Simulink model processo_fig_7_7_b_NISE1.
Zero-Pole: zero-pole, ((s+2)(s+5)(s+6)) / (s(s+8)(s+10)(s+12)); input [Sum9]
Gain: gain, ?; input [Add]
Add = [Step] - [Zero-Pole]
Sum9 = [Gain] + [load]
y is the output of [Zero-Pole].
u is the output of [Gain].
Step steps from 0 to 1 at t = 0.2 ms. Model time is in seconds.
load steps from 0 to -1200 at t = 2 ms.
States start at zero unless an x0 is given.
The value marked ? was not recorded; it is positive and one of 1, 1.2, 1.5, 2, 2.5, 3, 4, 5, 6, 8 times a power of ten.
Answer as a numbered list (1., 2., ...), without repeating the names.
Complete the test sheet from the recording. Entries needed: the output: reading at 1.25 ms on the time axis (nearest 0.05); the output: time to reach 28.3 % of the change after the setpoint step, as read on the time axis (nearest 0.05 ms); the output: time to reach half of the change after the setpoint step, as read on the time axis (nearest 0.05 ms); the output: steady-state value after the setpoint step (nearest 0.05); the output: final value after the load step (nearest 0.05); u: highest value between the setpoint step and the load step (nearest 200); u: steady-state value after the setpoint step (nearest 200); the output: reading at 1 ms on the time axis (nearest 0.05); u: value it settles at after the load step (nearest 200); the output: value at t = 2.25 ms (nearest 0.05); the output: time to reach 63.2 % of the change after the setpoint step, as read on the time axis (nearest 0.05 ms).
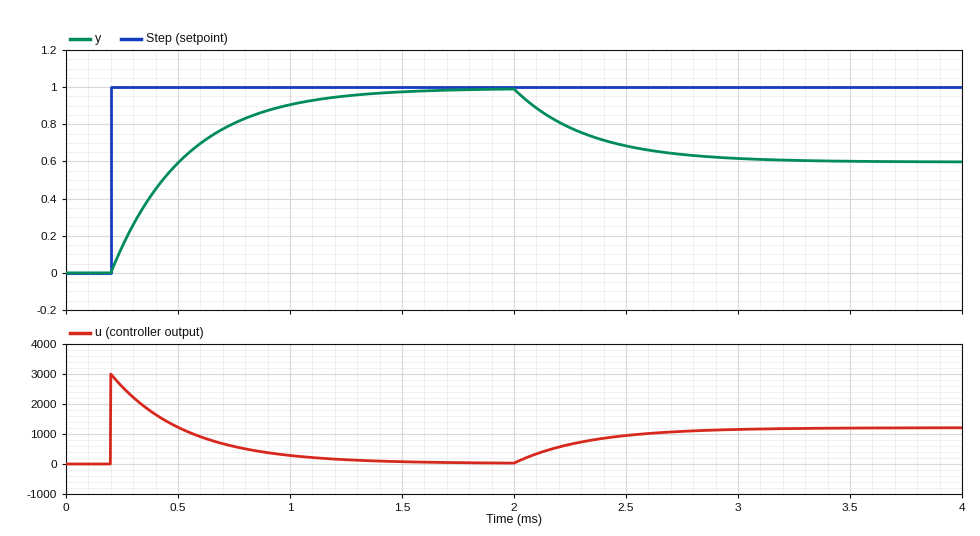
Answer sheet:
1. 0.95
2. 0.30 ms
3. 0.45 ms
4. 1.00
5. 0.60
6. 3000
7. 0
8. 0.90
9. 1200
10. 0.80
11. 0.55 ms
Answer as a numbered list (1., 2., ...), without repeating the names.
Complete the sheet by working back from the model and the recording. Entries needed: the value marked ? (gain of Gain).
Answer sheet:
1. 3000
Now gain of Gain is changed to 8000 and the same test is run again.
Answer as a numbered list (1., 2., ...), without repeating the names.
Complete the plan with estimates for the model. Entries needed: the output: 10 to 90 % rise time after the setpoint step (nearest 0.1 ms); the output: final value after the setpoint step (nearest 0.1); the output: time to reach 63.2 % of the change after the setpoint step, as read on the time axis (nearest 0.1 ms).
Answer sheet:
1. 0.3 ms
2. 1.0
3. 0.3 ms
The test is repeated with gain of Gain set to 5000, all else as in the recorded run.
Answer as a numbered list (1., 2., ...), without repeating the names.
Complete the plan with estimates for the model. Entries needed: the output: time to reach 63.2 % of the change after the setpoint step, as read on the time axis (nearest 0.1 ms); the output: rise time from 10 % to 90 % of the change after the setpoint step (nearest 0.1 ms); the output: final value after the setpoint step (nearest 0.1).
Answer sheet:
1. 0.4 ms
2. 0.4 ms
3. 1.0
